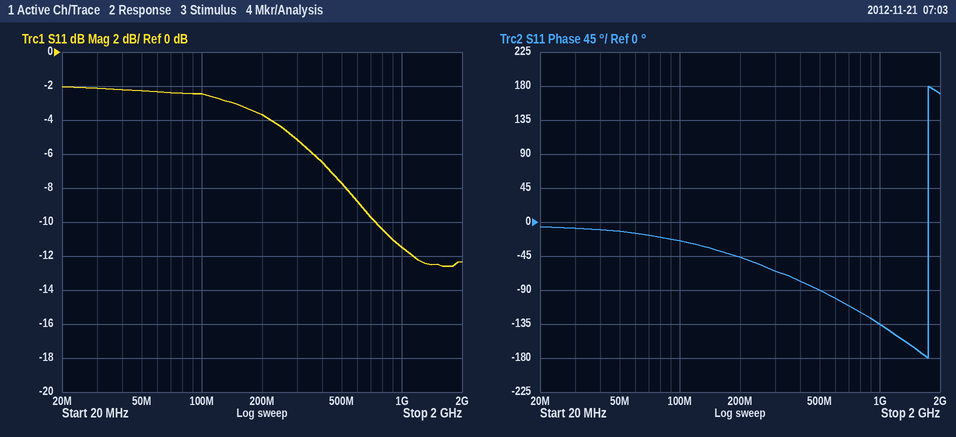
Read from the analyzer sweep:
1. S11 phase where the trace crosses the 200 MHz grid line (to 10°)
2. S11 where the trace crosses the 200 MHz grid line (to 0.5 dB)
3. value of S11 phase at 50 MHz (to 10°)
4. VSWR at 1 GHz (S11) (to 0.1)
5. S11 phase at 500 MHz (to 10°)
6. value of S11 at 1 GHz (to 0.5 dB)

-50°
-3.5 dB
-10°
1.7
-90°
-11.5 dB
